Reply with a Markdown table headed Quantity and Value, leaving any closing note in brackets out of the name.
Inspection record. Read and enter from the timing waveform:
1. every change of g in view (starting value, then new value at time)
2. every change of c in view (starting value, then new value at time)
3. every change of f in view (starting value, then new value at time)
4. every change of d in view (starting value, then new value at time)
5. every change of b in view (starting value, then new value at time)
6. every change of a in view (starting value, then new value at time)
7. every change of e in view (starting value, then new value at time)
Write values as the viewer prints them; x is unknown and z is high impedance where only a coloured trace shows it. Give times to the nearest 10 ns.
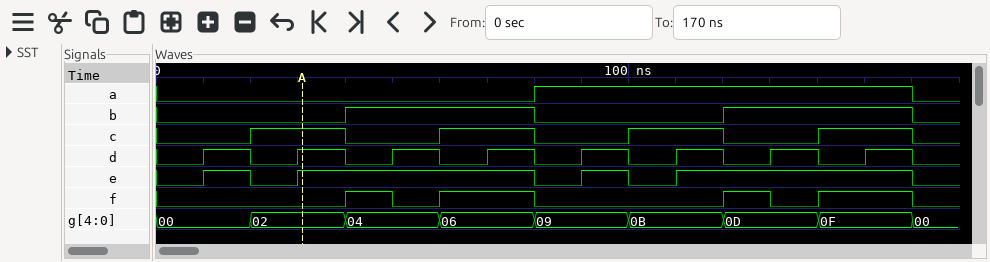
| Quantity | Value |
|---|---|
| every change of g in view | 00, 02 at 20 ns, 04 at 40 ns, 06 at 60 ns, 09 at 80 ns, 0B at 100 ns, 0D at 120 ns, 0F at 140 ns, 00 at 160 ns |
| every change of c in view | 0, 1 at 20 ns, 0 at 40 ns, 1 at 60 ns, 0 at 80 ns, 1 at 100 ns, 0 at 120 ns, 1 at 140 ns, 0 at 160 ns |
| every change of f in view | 0, 1 at 40 ns, 0 at 50 ns, 1 at 60 ns, 0 at 80 ns, 1 at 120 ns, 0 at 130 ns, 1 at 140 ns, 0 at 160 ns |
| every change of d in view | 0, 1 at 10 ns, 0 at 20 ns, 1 at 30 ns, 0 at 40 ns, 1 at 50 ns, 0 at 60 ns, 1 at 70 ns, 0 at 80 ns, 1 at 90 ns, 0 at 100 ns, 1 at 110 ns, 0 at 120 ns, 1 at 130 ns, 0 at 140 ns, 1 at 150 ns, 0 at 160 ns |
| every change of b in view | 0, 1 at 40 ns, 0 at 80 ns, 1 at 120 ns, 0 at 160 ns |
| every change of a in view | 0, 1 at 80 ns, 0 at 160 ns |
| every change of e in view | 0, 1 at 10 ns, 0 at 20 ns, 1 at 30 ns, 0 at 80 ns, 1 at 90 ns, 0 at 100 ns, 1 at 110 ns, 0 at 160 ns |
